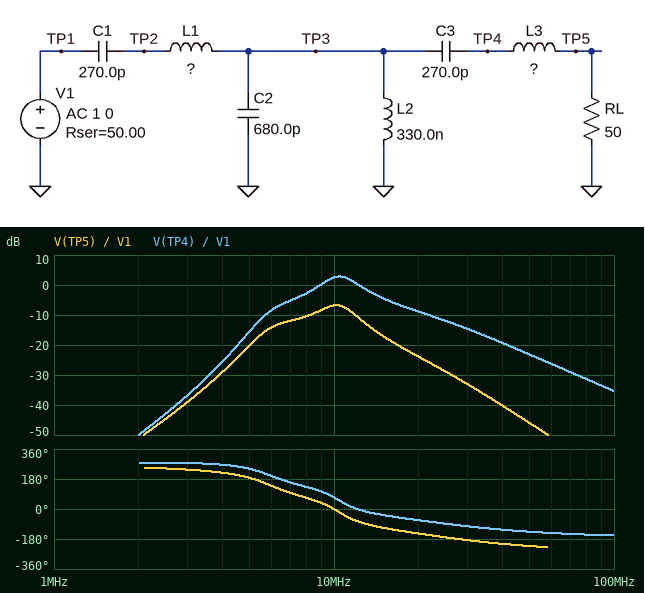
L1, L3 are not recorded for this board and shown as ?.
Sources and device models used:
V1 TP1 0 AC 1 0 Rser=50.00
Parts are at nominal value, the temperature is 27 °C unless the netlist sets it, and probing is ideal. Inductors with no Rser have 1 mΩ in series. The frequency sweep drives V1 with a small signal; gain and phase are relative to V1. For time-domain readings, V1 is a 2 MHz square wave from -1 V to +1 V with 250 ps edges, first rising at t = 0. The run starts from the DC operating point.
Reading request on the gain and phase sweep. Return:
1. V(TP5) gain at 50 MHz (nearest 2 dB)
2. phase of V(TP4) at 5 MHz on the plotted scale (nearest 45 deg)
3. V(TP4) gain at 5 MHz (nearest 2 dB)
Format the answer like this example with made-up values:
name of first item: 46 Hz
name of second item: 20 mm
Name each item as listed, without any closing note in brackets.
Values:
V(TP5) gain at 50 MHz: -46 dB
phase of V(TP4) at 5 MHz on the plotted scale: 225 deg
V(TP4) gain at 5 MHz: -16 dB
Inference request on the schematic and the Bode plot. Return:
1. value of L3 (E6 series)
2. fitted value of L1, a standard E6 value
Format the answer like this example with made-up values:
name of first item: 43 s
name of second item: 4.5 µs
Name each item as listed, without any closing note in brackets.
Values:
value of L3: 2.2 µH
fitted value of L1, a standard E6 value: 220 nH
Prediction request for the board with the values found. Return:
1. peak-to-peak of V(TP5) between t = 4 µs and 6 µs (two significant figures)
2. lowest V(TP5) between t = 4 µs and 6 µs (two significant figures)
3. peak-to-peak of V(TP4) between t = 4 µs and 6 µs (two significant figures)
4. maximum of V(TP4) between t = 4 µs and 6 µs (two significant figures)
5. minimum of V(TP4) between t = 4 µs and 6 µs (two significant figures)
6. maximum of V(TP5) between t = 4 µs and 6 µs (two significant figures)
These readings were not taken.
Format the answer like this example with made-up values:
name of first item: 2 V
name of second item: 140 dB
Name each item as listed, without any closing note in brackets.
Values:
peak-to-peak of V(TP5) between t = 4 µs and 6 µs: 450 mV
lowest V(TP5) between t = 4 µs and 6 µs: -230 mV
peak-to-peak of V(TP4) between t = 4 µs and 6 µs: 1.2 V
maximum of V(TP4) between t = 4 µs and 6 µs: 620 mV
minimum of V(TP4) between t = 4 µs and 6 µs: -620 mV
maximum of V(TP5) between t = 4 µs and 6 µs: 230 mV
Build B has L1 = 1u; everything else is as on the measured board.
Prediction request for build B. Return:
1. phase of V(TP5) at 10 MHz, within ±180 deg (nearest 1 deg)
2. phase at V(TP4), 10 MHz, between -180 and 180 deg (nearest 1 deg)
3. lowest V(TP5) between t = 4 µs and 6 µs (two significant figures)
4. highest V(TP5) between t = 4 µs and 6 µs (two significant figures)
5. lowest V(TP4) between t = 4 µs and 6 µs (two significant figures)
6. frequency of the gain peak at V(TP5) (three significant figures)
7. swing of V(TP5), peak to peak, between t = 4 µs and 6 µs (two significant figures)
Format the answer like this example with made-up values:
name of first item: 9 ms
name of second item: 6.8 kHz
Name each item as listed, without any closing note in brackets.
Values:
phase of V(TP5) at 10 MHz, within ±180 deg: -30 deg
phase at V(TP4), 10 MHz, between -180 and 180 deg: 40 deg
lowest V(TP5) between t = 4 µs and 6 µs: -240 mV
highest V(TP5) between t = 4 µs and 6 µs: 240 mV
lowest V(TP4) between t = 4 µs and 6 µs: -630 mV
frequency of the gain peak at V(TP5): 12.5 MHz
swing of V(TP5), peak to peak, between t = 4 µs and 6 µs: 490 mV
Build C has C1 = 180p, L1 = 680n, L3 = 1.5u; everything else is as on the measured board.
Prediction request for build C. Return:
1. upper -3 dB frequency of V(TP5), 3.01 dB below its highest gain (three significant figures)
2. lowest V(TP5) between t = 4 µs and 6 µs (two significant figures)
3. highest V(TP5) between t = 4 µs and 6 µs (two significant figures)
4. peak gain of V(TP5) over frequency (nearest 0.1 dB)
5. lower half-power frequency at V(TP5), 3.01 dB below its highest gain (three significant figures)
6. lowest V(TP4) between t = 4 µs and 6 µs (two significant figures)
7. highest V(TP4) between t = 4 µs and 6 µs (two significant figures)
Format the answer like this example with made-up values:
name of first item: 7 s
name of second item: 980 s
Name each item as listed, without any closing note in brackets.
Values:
upper -3 dB frequency of V(TP5), 3.01 dB below its highest gain: 13.3 MHz
lowest V(TP5) between t = 4 µs and 6 µs: -240 mV
highest V(TP5) between t = 4 µs and 6 µs: 240 mV
peak gain of V(TP5) over frequency: -6.0 dB
lower half-power frequency at V(TP5), 3.01 dB below its highest gain: 8.06 MHz
lowest V(TP4) between t = 4 µs and 6 µs: -540 mV
highest V(TP4) between t = 4 µs and 6 µs: 540 mV
